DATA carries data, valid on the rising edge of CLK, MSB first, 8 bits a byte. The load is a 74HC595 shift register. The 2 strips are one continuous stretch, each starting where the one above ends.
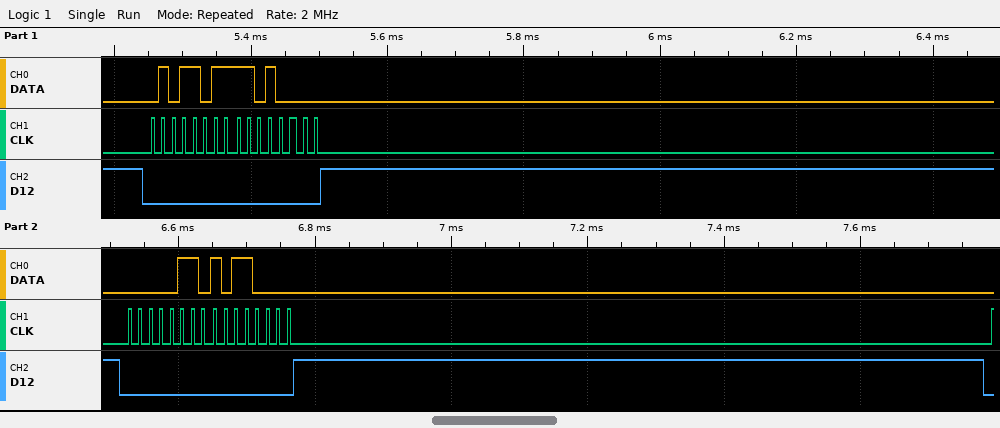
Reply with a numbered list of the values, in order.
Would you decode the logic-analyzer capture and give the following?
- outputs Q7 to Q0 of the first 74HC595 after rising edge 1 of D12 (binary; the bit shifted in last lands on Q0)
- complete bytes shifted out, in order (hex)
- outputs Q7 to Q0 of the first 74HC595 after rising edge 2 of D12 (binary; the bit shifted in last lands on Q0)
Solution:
1. 11010000
2. 5B D0 06 B0
3. 10110000
